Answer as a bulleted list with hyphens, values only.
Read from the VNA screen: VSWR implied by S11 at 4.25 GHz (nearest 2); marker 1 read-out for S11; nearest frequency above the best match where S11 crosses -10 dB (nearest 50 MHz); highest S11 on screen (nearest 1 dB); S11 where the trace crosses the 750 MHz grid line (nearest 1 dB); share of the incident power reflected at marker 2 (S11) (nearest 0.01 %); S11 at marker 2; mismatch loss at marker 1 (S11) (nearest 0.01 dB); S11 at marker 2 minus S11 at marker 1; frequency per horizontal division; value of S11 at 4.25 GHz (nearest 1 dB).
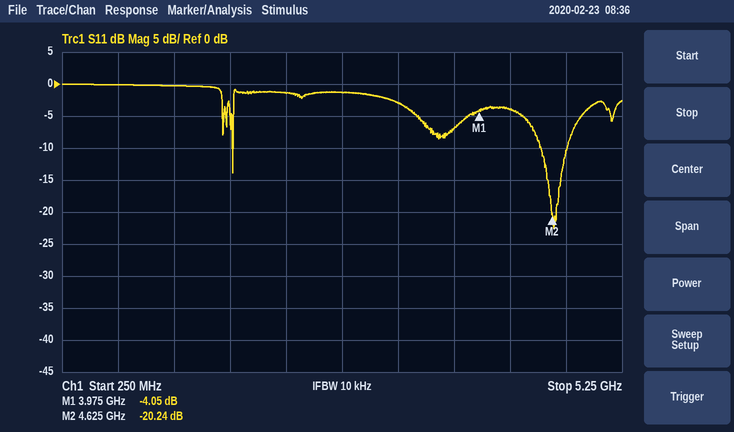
- 4
- -4.05 dB
- 4.75 GHz
- 0 dB
- 0 dB
- 0.95 %
- -20.24 dB
- 2.17 dB
- -16.19 dB
- 500 MHz
- -4 dB
